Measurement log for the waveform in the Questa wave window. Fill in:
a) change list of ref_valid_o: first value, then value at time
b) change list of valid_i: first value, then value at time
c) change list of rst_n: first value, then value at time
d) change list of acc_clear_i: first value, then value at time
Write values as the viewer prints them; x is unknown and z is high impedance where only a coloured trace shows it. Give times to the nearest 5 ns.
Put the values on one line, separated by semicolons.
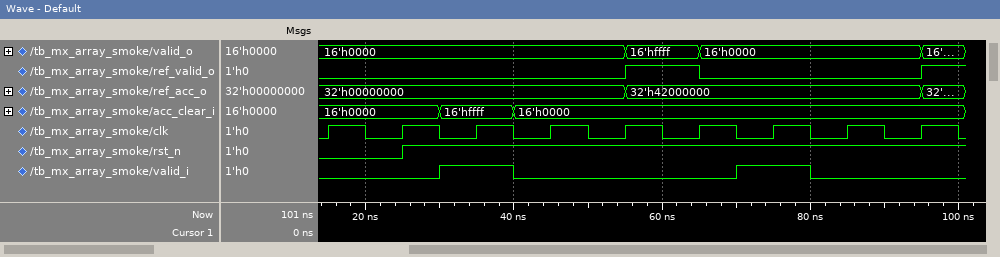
0, 1 at 55 ns, 0 at 65 ns, 1 at 95 ns; 0, 1 at 30 ns, 0 at 40 ns, 1 at 70 ns, 0 at 80 ns; 0, 1 at 25 ns; 16'h0000, 16'hffff at 30 ns, 16'h0000 at 40 ns
